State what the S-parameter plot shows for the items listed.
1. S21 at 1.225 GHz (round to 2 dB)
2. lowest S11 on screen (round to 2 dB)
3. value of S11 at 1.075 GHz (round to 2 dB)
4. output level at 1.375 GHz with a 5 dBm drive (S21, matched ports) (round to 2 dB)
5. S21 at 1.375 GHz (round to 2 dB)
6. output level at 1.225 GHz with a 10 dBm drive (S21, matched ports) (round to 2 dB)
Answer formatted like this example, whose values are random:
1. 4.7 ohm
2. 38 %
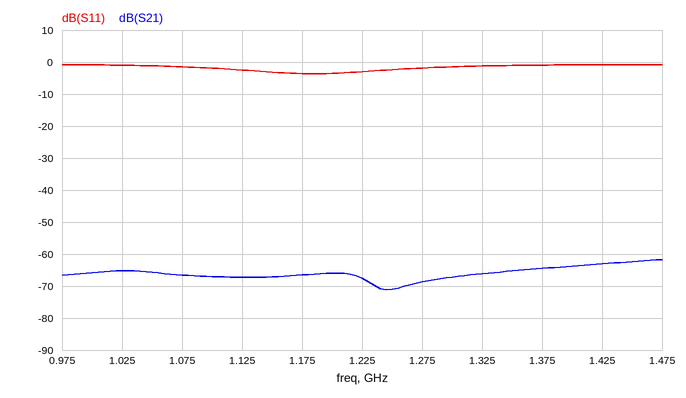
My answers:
1. -68 dB
2. -4 dB
3. -2 dB
4. -60 dBm
5. -64 dB
6. -58 dBm
